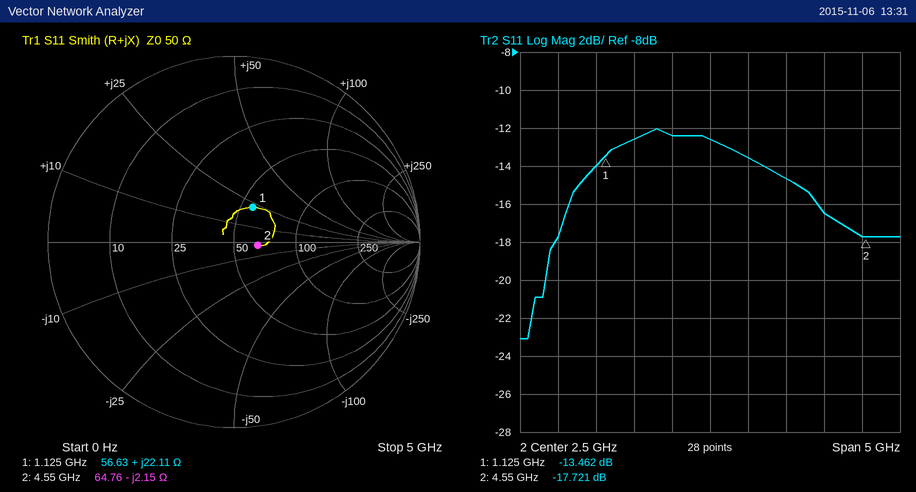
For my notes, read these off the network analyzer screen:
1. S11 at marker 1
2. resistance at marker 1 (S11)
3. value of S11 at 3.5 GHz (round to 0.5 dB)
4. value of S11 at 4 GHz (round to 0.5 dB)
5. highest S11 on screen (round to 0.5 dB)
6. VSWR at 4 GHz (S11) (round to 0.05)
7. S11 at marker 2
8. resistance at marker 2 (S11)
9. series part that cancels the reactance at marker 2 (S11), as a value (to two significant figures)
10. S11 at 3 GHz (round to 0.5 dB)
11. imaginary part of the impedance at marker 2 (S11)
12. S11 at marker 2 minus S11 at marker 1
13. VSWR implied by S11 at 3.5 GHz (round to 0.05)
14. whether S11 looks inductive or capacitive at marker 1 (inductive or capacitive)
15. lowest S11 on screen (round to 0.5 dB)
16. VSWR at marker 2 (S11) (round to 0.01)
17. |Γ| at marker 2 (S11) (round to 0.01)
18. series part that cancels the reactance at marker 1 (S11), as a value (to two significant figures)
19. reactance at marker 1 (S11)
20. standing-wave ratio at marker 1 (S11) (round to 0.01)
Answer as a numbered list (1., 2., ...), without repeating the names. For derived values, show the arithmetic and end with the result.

1. -13.462 dB
2. 56.63 Ω
3. -14.5 dB
4. -16.5 dB
5. -12.0 dB
6. |Γ| = 10^(-16.5/20) = 0.1496; VSWR = (1 + 0.1496)/(1 − 0.1496) ≈ 1.35
7. -17.721 dB
8. 64.76 Ω
9. L = 2.15 Ω/(2π × 4.55 GHz) ≈ 75 pH
10. -13.5 dB
11. -2.15 Ω
12. -17.721 − (-13.462) = -4.259 dB
13. |Γ| = 10^(-14.5/20) = 0.1884; VSWR = (1 + 0.1884)/(1 − 0.1884) ≈ 1.46, so 1.45 to the nearest 0.05
14. inductive
15. -23.0 dB
16. (1 + 0.1300)/(1 − 0.1300) ≈ 1.30
17. 0.13
18. C = 1/(2π × 1.125 GHz × 22.11 Ω) ≈ 6.4 pF
19. +22.11 Ω
20. 1.54
